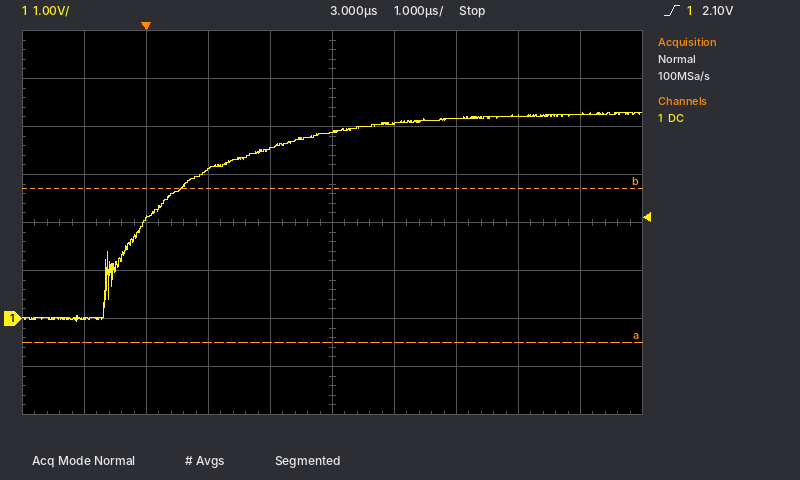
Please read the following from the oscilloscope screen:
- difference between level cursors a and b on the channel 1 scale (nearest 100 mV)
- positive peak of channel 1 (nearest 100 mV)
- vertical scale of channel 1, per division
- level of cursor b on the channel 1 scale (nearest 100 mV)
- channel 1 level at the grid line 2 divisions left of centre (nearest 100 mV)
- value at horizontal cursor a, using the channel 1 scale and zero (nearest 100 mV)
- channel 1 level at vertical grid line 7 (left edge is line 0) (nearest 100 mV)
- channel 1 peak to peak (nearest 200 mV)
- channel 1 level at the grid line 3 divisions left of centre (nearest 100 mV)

3.2 V
4.3 V
1 V
2.7 V
3.1 V
-500 mV
4.2 V
4.4 V
2.1 V
